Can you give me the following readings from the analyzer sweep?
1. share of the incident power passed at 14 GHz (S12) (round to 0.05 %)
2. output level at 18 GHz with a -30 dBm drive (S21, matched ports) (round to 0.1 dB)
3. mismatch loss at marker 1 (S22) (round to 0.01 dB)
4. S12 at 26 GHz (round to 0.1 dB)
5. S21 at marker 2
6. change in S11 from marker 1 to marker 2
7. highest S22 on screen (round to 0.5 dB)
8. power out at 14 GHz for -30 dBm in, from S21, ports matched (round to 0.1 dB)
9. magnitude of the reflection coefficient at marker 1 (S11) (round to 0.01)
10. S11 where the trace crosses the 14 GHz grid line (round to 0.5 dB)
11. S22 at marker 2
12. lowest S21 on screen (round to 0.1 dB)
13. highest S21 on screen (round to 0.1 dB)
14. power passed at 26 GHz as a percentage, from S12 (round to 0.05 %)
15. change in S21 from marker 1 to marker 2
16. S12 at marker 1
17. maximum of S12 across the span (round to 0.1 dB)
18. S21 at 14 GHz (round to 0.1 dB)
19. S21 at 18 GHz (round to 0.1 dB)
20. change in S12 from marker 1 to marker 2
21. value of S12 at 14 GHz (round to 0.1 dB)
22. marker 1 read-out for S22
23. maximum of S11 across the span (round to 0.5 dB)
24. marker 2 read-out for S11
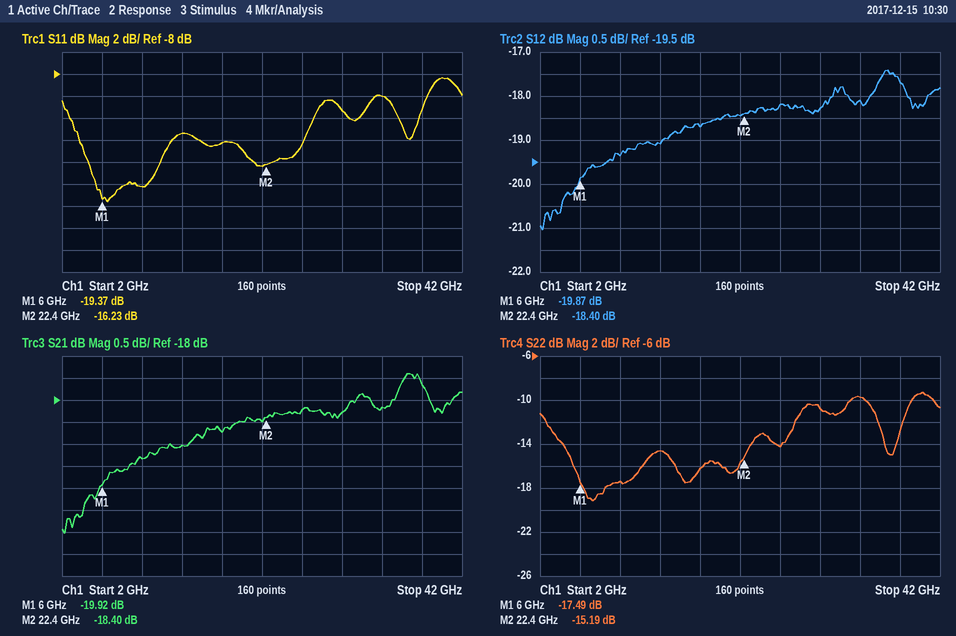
1.25 %
-48.7 dBm
0.08 dB
-18.2 dB
-18.40 dB
3.14 dB
-9.5 dB
-49.0 dBm
0.11
-13.5 dB
-15.19 dB
-21.0 dB
-17.4 dB
1.50 %
1.52 dB
-19.87 dB
-17.4 dB
-19.0 dB
-18.7 dB
1.47 dB
-19.1 dB
-17.49 dB
-8.5 dB
-16.23 dB
